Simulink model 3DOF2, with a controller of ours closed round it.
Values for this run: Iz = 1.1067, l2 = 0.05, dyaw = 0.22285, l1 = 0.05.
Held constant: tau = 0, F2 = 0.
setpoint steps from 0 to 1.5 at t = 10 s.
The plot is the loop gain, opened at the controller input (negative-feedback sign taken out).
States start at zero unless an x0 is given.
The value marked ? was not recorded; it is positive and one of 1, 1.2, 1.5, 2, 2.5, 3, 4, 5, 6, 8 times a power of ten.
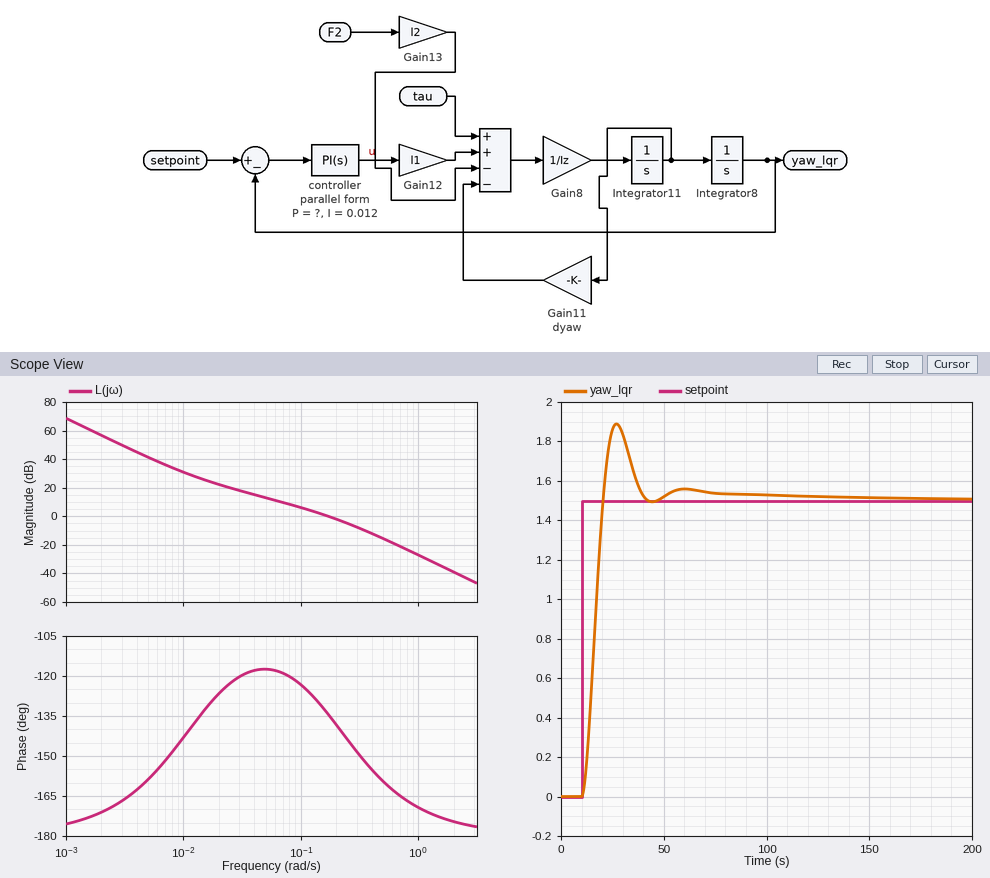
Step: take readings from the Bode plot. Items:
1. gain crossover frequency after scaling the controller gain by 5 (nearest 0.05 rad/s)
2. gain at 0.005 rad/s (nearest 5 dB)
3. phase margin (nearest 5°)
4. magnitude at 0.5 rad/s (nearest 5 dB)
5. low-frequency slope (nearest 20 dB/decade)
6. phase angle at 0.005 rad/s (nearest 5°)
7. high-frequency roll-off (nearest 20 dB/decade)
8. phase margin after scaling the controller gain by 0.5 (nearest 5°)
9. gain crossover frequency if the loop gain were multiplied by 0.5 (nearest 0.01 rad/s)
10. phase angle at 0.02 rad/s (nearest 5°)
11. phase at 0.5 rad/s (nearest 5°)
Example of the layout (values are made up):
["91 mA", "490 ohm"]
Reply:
["0.45 rad/s", "40 dB", "45°", "-15 dB", "-40 dB/decade", "-160°", "-40 dB/decade", "55°", "0.10 rad/s", "-125°", "-160°"]
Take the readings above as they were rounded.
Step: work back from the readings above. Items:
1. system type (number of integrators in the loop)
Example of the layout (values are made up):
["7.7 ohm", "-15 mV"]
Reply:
["2"]
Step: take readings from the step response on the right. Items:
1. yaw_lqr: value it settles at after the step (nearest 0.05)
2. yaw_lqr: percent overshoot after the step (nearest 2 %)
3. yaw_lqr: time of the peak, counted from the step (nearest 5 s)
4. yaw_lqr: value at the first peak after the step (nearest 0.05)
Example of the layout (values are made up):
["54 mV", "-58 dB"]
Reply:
["1.50", "26 %", "15 s", "1.90"]
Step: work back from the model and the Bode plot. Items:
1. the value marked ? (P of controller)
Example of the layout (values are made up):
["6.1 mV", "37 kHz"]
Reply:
["1"]
